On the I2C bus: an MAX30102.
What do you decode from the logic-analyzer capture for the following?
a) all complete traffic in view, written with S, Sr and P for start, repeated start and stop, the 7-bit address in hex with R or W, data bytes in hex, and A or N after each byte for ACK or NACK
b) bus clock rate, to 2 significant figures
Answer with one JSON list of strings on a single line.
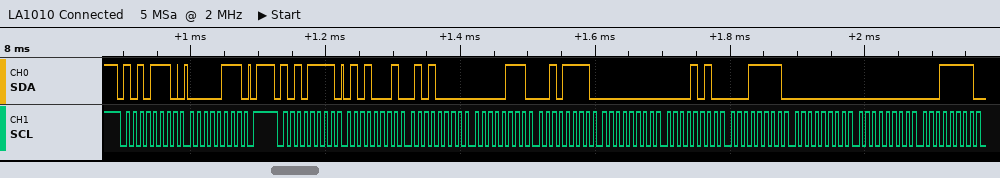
["S 57W A 07 A P S 57R A 51 A 50 A 07 A 2F A 00 A 0A A 1F A 00 A 00 A 1F A", "100 kHz"]
